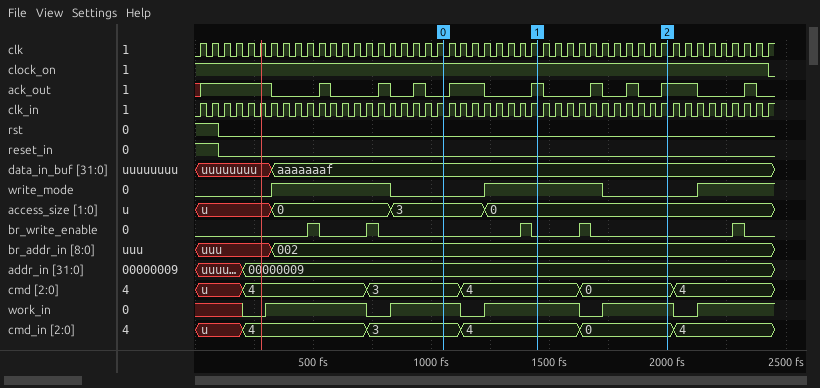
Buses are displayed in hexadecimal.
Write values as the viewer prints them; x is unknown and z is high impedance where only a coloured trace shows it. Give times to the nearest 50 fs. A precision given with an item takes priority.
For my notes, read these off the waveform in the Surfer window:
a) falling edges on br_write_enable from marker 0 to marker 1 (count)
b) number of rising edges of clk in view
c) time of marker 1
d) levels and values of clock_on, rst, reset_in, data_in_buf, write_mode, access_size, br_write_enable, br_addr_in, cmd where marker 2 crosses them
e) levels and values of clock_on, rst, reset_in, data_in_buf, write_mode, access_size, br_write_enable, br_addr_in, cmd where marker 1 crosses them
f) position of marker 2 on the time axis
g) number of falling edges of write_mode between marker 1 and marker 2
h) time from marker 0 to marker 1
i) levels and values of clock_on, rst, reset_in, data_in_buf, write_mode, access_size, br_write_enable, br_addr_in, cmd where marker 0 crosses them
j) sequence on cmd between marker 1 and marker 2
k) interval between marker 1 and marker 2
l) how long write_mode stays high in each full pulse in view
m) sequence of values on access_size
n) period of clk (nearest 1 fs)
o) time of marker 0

1
49
1450 fs
clock_on=1, rst=0, reset_in=0, data_in_buf=aaaaaaaf, write_mode=0, access_size=0, br_write_enable=0, br_addr_in=002, cmd=0
clock_on=1, rst=0, reset_in=0, data_in_buf=aaaaaaaf, write_mode=1, access_size=0, br_write_enable=0, br_addr_in=002, cmd=4
2000 fs
1
400 fs
clock_on=1, rst=0, reset_in=0, data_in_buf=aaaaaaaf, write_mode=0, access_size=3, br_write_enable=0, br_addr_in=002, cmd=3
4, 0
550 fs
500 fs, 500 fs
u, 0, 3, 0
50 fs
1050 fs
